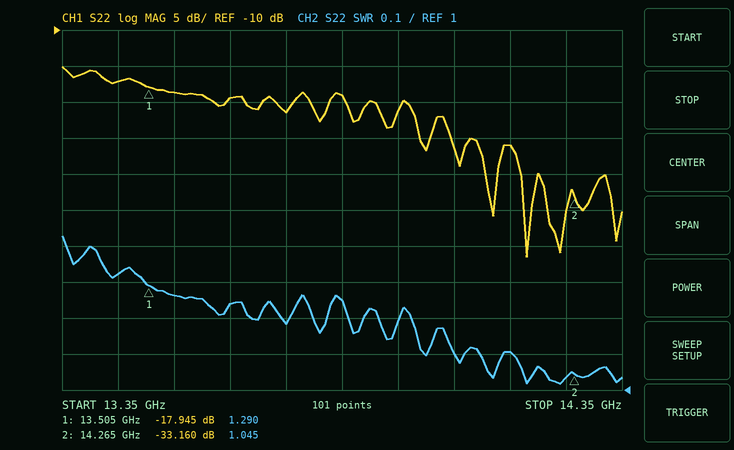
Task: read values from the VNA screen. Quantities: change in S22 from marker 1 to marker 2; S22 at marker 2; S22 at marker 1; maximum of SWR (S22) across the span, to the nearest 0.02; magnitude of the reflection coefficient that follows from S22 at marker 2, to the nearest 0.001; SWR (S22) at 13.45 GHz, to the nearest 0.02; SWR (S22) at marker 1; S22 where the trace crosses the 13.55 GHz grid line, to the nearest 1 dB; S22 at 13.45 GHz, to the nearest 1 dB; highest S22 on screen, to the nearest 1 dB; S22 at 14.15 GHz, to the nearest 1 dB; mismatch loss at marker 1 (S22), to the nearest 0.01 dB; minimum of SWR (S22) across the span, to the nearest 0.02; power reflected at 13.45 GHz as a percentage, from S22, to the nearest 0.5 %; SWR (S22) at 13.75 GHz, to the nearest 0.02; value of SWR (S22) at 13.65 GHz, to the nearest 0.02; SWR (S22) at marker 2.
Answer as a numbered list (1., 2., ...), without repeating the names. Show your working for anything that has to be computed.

1. -33.16 − (-17.945) = -15.215 dB
2. -33.160 dB
3. -17.945 dB
4. 1.42
5. 10^(-33.16/20) ≈ 0.022
6. 1.32
7. 1.290
8. -19 dB
9. -17 dB
10. -15 dB
11. -26 dB
12. −10 log10(1 − 10^(-17.945/10)) ≈ 0.07 dB
13. 1.02
14. 10^(-17/10) ≈ 2.0 %
15. 1.18
16. 1.24
17. 1.045
